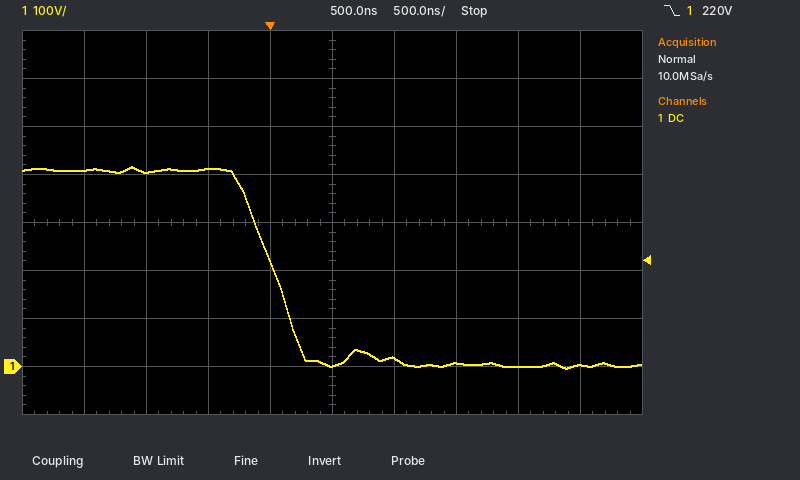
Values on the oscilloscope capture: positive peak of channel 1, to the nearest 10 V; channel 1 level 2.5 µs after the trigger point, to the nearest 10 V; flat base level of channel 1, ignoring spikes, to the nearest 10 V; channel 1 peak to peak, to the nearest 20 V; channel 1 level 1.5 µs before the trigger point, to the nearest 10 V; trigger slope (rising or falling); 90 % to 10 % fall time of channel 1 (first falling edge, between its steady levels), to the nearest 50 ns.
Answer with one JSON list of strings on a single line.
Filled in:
["420 V", "0 V", "0 V", "420 V", "410 V", "falling", "450 ns"]
